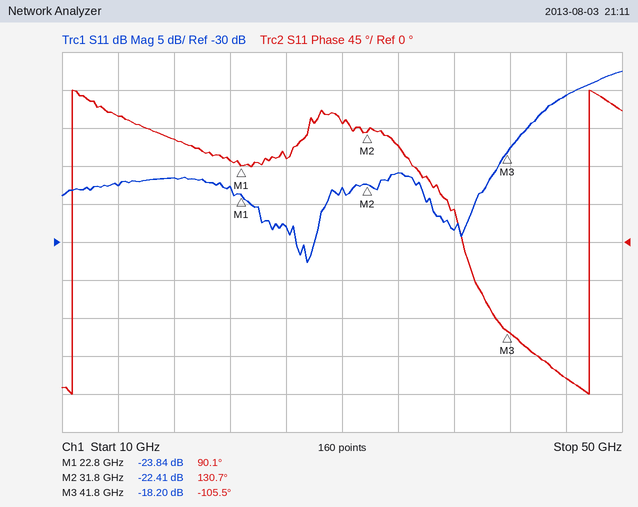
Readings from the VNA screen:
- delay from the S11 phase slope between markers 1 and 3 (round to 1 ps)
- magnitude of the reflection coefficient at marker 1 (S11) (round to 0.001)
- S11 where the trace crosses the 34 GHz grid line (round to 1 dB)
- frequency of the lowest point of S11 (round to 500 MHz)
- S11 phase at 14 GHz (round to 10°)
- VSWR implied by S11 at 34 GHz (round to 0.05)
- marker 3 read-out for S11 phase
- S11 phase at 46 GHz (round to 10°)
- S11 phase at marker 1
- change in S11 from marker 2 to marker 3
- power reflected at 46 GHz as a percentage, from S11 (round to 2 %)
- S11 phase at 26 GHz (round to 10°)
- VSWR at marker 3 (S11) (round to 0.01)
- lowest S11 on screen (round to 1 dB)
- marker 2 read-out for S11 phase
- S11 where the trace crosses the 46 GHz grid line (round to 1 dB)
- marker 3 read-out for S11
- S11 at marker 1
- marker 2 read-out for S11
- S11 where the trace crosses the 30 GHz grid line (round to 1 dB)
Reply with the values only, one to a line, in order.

29 ps
0.064
-21 dB
27.5 GHz
150°
1.20
-105.5°
-160°
90.1°
4.21 dB
8 %
100°
1.28
-33 dB
130.7°
-11 dB
-18.20 dB
-23.84 dB
-22.41 dB
-23 dB
